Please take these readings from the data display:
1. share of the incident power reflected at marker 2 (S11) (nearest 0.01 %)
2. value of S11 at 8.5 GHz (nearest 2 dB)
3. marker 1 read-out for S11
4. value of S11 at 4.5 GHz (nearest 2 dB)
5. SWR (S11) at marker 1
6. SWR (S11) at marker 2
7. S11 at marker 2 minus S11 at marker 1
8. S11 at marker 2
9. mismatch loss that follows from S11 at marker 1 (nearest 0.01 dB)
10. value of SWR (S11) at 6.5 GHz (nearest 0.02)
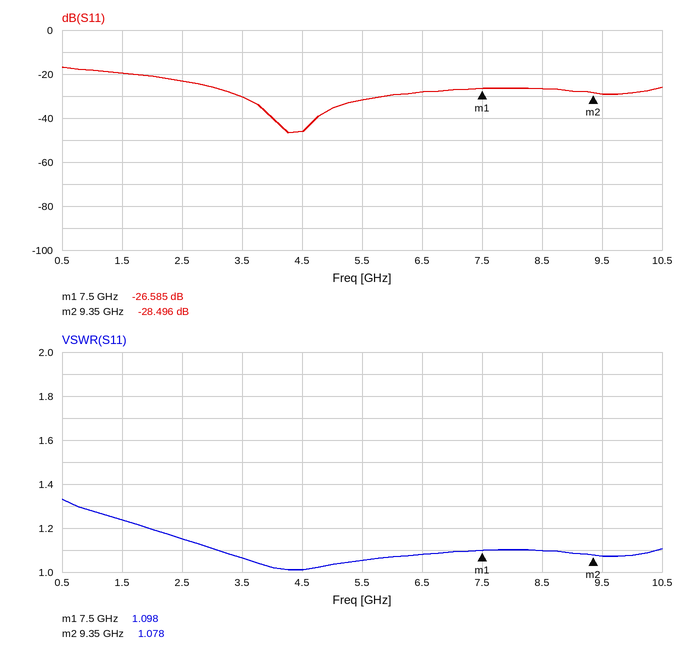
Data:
0.14 %
-26 dB
-26.585 dB
-46 dB
1.098
1.078
-1.911 dB
-28.496 dB
0.01 dB
1.08
